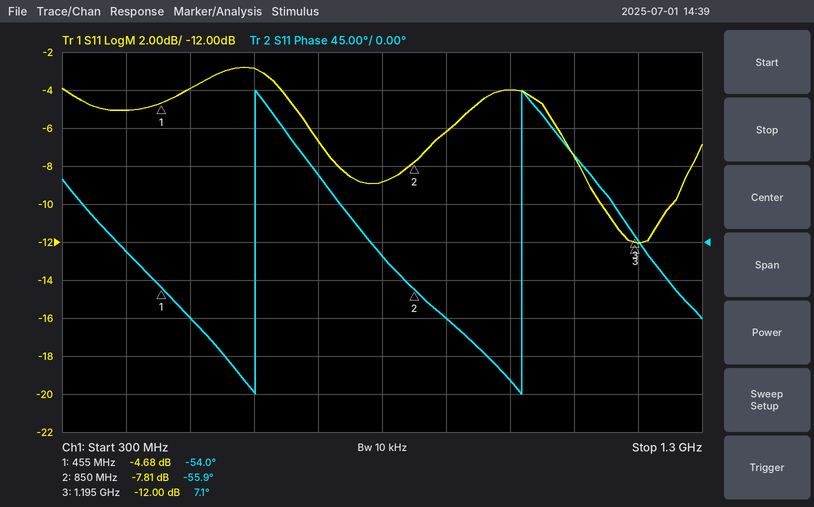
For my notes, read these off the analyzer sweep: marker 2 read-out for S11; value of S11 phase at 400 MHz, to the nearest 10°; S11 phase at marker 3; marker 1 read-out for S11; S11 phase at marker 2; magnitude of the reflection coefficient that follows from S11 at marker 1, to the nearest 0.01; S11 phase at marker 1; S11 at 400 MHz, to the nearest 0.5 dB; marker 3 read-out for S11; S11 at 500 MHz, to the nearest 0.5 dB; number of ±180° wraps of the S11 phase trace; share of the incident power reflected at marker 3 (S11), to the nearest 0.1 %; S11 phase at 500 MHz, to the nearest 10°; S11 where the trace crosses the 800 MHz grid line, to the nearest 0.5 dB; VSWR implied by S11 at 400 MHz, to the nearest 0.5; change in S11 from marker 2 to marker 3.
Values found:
-7.81 dB
-10°
7.1°
-4.68 dB
-55.9°
0.58
-54.0°
-5.0 dB
-12.00 dB
-4.0 dB
2
6.3 %
-90°
-9.0 dB
3.5
-4.19 dB
